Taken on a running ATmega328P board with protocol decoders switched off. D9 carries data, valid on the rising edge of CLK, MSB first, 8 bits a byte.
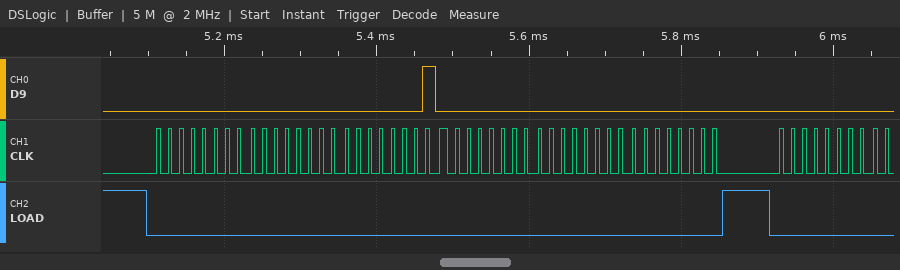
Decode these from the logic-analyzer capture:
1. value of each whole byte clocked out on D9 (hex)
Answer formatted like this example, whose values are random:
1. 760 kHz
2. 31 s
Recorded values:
1. 00 00 01 00 00 00 00
